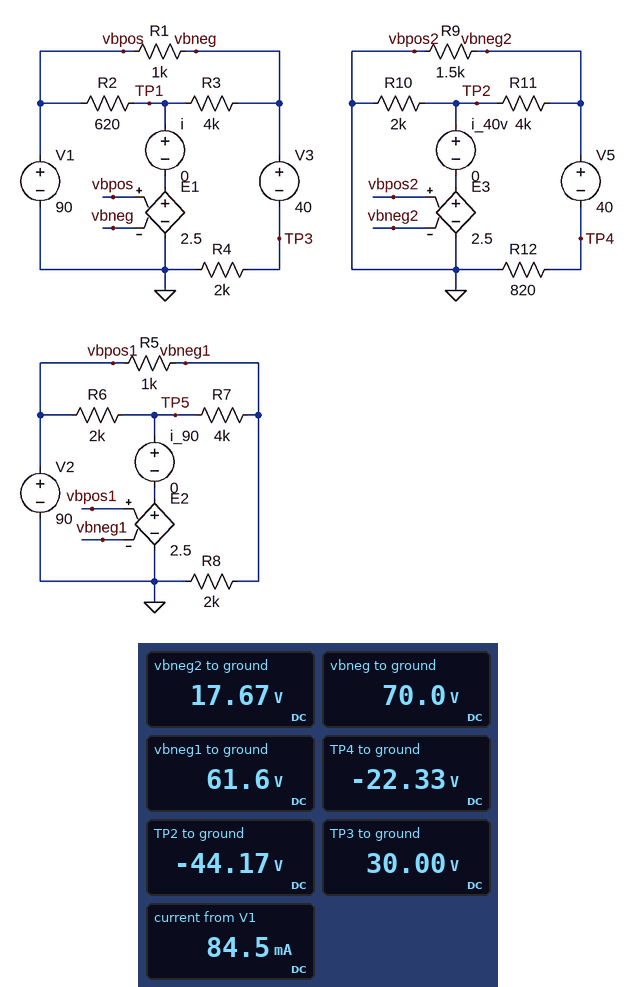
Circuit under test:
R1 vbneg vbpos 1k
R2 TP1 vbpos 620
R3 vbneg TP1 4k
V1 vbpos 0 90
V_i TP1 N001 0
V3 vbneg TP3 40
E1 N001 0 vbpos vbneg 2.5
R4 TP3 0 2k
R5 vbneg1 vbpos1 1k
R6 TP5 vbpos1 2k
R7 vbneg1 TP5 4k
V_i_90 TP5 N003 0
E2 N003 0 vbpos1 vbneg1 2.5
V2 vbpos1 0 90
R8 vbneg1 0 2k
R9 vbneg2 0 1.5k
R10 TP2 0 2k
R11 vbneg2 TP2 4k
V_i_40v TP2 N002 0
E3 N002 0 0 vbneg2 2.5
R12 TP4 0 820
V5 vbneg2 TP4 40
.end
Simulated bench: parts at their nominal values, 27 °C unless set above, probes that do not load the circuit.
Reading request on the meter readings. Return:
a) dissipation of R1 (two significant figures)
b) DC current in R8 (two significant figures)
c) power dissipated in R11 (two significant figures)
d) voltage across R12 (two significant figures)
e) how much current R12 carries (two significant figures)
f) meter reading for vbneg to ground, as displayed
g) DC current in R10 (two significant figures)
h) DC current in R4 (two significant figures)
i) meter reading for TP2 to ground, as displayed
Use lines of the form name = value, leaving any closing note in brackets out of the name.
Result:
dissipation of R1 = 400 mW
DC current in R8 = 31 mA
power dissipated in R11 = 960 mW
voltage across R12 = 22 V
how much current R12 carries = 27 mA
meter reading for vbneg to ground, as displayed = 70.0 V
DC current in R10 = 22 mA
DC current in R4 = 15 mA
meter reading for TP2 to ground, as displayed = -44.17 V
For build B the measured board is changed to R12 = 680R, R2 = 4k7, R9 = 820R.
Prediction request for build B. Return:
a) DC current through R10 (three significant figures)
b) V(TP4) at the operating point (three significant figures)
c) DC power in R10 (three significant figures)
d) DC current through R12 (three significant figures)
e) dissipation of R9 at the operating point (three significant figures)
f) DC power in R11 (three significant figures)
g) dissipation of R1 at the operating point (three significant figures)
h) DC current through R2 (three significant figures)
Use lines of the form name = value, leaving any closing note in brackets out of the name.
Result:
DC current through R10 = 20.6 mA
V(TP4) at the operating point = -23.5 V
DC power in R10 = 851 mW
DC current through R12 = 34.6 mA
dissipation of R9 at the operating point = 332 mW
DC power in R11 = 834 mW
dissipation of R1 at the operating point = 400 mW
DC current through R2 = 8.51 mA
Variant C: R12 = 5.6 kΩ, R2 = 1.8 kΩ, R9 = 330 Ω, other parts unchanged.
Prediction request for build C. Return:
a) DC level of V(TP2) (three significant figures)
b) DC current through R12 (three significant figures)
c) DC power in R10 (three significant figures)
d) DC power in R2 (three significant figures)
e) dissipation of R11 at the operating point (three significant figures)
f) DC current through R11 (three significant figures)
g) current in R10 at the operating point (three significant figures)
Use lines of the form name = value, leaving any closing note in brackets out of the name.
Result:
DC level of V(TP2) = -4.37 V
DC current through R12 = 6.83 mA
DC power in R10 = 9.56 mW
DC power in R2 = 889 mW
dissipation of R11 at the operating point = 9.37 mW
DC current through R11 = 1.53 mA
current in R10 at the operating point = 2.19 mA
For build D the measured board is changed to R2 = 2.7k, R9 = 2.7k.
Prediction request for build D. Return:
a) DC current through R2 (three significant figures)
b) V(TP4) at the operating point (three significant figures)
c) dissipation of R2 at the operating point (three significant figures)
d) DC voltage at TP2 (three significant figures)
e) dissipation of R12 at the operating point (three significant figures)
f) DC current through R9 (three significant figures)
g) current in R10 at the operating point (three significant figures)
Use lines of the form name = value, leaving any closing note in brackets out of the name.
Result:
DC current through R2 = 14.8 mA
V(TP4) at the operating point = -20.2 V
dissipation of R2 at the operating point = 593 mW
DC voltage at TP2 = -49.5 V
dissipation of R12 at the operating point = 498 mW
DC current through R9 = 7.33 mA
current in R10 at the operating point = 24.7 mA
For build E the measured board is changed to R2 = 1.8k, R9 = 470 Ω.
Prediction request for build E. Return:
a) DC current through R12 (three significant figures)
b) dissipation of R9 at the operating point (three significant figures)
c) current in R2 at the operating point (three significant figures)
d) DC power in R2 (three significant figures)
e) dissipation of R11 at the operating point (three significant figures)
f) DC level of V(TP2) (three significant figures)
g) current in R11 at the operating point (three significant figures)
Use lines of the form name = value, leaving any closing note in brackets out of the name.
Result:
DC current through R12 = 34.7 mA
dissipation of R9 at the operating point = 284 mW
current in R2 at the operating point = 22.2 mA
DC power in R2 = 889 mW
dissipation of R11 at the operating point = 409 mW
DC level of V(TP2) = -28.9 V
current in R11 at the operating point = 10.1 mA
